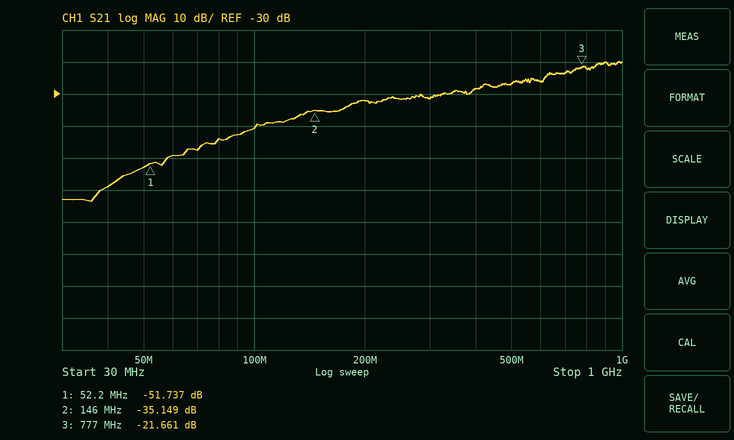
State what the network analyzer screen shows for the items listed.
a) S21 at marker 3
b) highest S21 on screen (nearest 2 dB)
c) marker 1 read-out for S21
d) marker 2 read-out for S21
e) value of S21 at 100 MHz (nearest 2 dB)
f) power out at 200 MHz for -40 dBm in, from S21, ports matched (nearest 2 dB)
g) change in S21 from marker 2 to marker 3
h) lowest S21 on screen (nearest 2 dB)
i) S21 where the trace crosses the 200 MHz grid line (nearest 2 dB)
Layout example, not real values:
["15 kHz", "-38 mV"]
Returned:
["-21.661 dB", "-20 dB", "-51.737 dB", "-35.149 dB", "-40 dB", "-72 dBm", "13.488 dB", "-64 dB", "-32 dB"]
